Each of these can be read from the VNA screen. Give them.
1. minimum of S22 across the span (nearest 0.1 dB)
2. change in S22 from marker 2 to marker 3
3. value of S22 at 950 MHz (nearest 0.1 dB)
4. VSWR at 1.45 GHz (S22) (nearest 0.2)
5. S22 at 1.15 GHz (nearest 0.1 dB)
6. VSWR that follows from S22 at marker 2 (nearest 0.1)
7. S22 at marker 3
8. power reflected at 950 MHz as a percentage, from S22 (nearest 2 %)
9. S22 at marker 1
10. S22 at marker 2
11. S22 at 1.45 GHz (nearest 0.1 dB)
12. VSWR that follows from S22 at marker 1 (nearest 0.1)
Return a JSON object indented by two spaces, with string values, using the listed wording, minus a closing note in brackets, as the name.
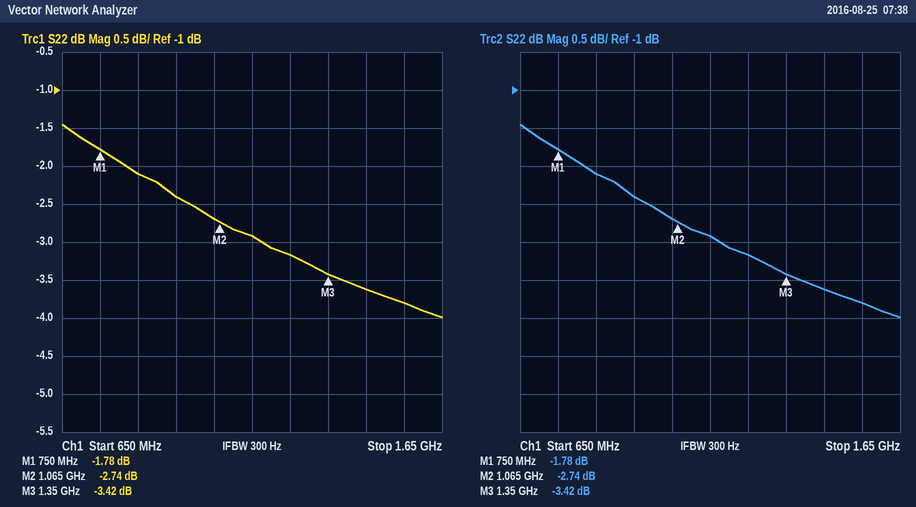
{
  "minimum of S22 across the span": "-4.0 dB",
  "change in S22 from marker 2 to marker 3": "-0.68 dB",
  "value of S22 at 950 MHz": "-2.4 dB",
  "VSWR at 1.45 GHz (S22)": "4.8",
  "S22 at 1.15 GHz": "-2.9 dB",
  "VSWR that follows from S22 at marker 2": "6.4",
  "S22 at marker 3": "-3.42 dB",
  "power reflected at 950 MHz as a percentage, from S22": "58 %",
  "S22 at marker 1": "-1.78 dB",
  "S22 at marker 2": "-2.74 dB",
  "S22 at 1.45 GHz": "-3.6 dB",
  "VSWR that follows from S22 at marker 1": "9.8"
}
